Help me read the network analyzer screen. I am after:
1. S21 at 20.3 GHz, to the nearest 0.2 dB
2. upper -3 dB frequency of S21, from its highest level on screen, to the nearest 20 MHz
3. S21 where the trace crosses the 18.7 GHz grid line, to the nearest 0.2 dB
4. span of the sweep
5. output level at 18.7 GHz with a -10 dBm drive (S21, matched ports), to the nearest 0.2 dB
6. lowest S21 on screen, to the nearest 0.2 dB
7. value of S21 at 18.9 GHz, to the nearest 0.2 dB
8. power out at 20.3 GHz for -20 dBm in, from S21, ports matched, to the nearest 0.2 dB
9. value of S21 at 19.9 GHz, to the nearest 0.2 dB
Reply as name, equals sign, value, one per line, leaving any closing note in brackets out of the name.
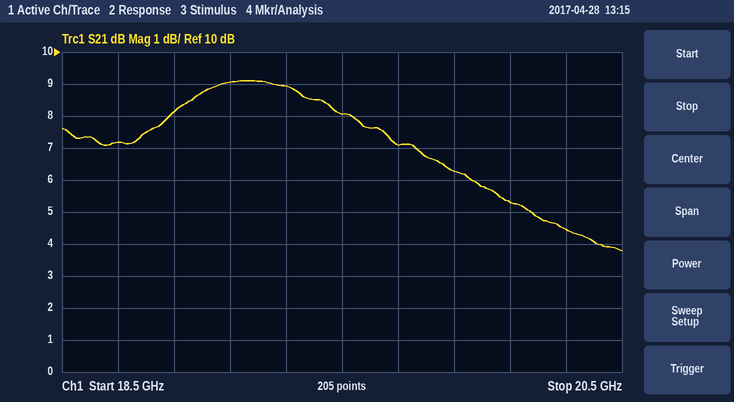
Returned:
S21 at 20.3 GHz, to the nearest 0.2 dB = 4.4 dB
upper -3 dB frequency of S21, from its highest level on screen, to the nearest 20 MHz = 19.94 GHz
S21 where the trace crosses the 18.7 GHz grid line, to the nearest 0.2 dB = 7.2 dB
span of the sweep = 2 GHz
output level at 18.7 GHz with a -10 dBm drive (S21, matched ports), to the nearest 0.2 dB = -2.8 dBm
lowest S21 on screen, to the nearest 0.2 dB = 3.8 dB
value of S21 at 18.9 GHz, to the nearest 0.2 dB = 8.2 dB
power out at 20.3 GHz for -20 dBm in, from S21, ports matched, to the nearest 0.2 dB = -15.6 dBm
value of S21 at 19.9 GHz, to the nearest 0.2 dB = 6.2 dB
